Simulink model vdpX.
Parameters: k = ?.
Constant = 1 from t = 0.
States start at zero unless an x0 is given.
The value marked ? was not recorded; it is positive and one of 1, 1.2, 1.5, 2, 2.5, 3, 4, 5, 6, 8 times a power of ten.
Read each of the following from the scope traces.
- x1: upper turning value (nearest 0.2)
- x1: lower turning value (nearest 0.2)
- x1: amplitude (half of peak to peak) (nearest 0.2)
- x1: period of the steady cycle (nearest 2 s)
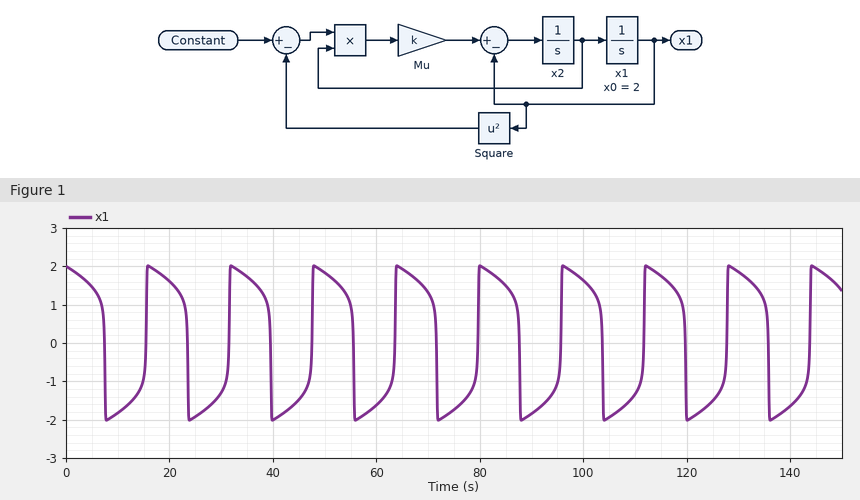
2.0
-2.0
2.0
16 s
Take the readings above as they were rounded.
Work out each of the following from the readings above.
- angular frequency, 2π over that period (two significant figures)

0.39 rad/s
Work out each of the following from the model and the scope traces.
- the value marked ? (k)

8
